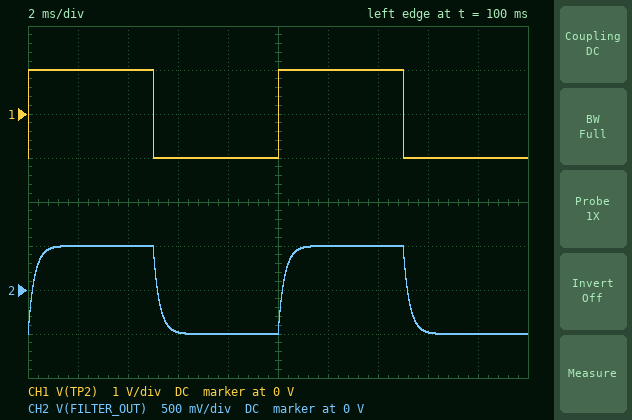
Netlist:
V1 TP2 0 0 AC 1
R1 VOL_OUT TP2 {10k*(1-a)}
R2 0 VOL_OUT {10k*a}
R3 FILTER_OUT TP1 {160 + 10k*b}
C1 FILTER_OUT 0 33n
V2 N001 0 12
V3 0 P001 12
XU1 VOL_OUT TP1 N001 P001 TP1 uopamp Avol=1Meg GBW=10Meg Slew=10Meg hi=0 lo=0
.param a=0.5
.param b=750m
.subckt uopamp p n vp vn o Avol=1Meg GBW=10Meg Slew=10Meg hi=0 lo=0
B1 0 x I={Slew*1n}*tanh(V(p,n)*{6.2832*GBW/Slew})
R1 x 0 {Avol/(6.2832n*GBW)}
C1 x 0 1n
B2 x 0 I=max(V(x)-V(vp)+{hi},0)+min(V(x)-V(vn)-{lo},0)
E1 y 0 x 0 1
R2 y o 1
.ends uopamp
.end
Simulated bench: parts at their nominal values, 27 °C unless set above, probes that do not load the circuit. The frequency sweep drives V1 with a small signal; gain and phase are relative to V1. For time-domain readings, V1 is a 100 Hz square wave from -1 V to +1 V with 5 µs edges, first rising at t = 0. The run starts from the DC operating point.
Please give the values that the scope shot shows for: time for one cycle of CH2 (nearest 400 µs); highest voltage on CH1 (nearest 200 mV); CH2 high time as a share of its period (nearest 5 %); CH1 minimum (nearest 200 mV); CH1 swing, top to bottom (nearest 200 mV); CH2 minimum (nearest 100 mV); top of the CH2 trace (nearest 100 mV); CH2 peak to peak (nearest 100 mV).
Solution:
10.0 ms
1.0 V
50 %
-1.0 V
2.0 V
-500 mV
500 mV
1.0 V
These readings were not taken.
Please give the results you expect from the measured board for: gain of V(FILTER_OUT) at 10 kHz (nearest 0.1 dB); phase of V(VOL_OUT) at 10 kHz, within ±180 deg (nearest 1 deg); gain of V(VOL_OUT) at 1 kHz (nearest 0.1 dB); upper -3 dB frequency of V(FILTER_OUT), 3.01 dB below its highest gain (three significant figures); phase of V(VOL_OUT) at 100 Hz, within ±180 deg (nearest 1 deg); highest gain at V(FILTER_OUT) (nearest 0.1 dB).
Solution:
-30.1 dB
0 deg
-6.0 dB
630 Hz
0 deg
-6.0 dB
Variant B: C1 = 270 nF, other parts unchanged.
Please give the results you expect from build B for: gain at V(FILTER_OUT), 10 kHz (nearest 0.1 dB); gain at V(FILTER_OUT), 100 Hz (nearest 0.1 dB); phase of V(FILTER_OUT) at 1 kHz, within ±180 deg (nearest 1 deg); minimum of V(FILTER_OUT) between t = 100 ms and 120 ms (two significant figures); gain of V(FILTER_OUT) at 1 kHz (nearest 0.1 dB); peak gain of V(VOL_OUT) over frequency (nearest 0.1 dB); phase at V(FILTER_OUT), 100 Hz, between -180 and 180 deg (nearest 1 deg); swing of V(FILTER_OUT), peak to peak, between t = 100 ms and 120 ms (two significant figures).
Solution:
-48.3 dB
-10.3 dB
-86 deg
-420 mV
-28.3 dB
-6.0 dB
-52 deg
840 mV
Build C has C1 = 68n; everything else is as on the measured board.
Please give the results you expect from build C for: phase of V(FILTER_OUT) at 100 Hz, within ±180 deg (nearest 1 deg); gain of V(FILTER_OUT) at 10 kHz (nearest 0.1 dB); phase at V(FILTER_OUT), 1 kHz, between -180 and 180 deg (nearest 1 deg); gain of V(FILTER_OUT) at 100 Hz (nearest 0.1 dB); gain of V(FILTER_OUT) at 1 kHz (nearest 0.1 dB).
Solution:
-18 deg
-36.3 dB
-73 deg
-6.5 dB
-16.7 dB
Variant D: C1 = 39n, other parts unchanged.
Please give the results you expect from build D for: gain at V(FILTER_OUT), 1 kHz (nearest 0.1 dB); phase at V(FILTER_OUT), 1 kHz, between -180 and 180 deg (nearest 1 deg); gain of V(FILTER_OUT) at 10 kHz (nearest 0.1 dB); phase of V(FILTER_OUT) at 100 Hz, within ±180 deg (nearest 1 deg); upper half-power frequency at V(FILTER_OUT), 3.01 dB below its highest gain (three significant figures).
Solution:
-12.6 dB
-62 deg
-31.5 dB
-11 deg
533 Hz
